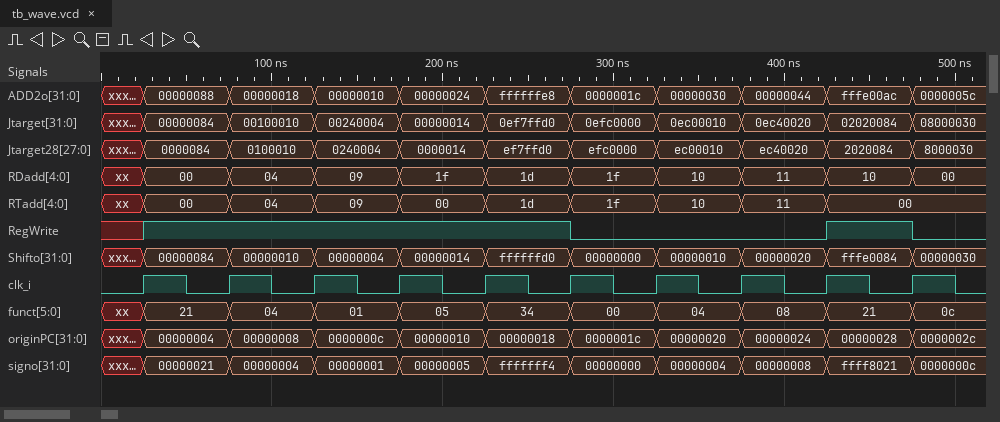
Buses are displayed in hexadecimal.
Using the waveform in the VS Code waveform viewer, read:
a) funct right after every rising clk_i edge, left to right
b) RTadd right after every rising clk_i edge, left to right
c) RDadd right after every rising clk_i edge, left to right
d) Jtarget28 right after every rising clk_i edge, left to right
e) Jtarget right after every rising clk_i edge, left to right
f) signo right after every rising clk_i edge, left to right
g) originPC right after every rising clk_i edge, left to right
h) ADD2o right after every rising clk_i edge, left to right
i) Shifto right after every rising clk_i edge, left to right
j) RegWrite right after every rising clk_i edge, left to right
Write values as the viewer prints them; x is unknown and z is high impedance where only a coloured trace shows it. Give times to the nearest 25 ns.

21, 04, 01, 05, 34, 00, 04, 08, 21, 0c
00, 04, 09, 00, 1d, 1f, 10, 11, 00, 00
00, 04, 09, 1f, 1d, 1f, 10, 11, 10, 00
0000084, 0100010, 0240004, 0000014, ef7ffd0, efc0000, ec00010, ec40020, 2020084, 8000030
00000084, 00100010, 00240004, 00000014, 0ef7ffd0, 0efc0000, 0ec00010, 0ec40020, 02020084, 08000030
00000021, 00000004, 00000001, 00000005, fffffff4, 00000000, 00000004, 00000008, ffff8021, 0000000c
00000004, 00000008, 0000000c, 00000010, 00000018, 0000001c, 00000020, 00000024, 00000028, 0000002c
00000088, 00000018, 00000010, 00000024, ffffffe8, 0000001c, 00000030, 00000044, fffe00ac, 0000005c
00000084, 00000010, 00000004, 00000014, ffffffd0, 00000000, 00000010, 00000020, fffe0084, 00000030
1 1 1 1 1 0 0 0 1 0
